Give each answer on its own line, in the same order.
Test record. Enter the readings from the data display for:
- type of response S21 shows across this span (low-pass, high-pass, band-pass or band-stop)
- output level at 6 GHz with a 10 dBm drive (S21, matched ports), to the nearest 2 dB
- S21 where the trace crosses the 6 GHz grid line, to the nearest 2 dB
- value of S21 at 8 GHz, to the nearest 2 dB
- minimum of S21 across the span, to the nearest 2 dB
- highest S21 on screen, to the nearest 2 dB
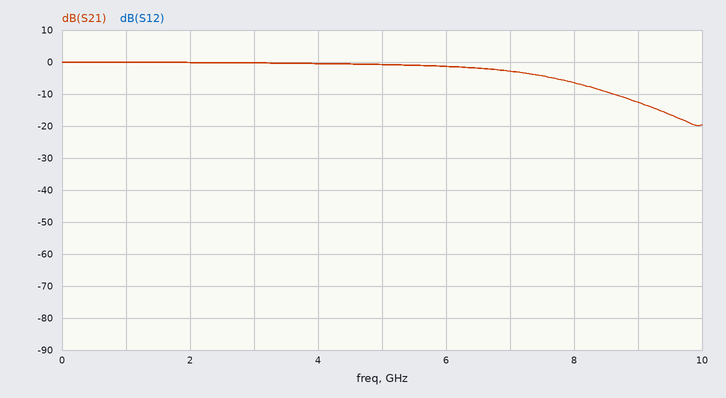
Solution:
low-pass
8 dBm
-2 dB
-6 dB
-20 dB
0 dB
